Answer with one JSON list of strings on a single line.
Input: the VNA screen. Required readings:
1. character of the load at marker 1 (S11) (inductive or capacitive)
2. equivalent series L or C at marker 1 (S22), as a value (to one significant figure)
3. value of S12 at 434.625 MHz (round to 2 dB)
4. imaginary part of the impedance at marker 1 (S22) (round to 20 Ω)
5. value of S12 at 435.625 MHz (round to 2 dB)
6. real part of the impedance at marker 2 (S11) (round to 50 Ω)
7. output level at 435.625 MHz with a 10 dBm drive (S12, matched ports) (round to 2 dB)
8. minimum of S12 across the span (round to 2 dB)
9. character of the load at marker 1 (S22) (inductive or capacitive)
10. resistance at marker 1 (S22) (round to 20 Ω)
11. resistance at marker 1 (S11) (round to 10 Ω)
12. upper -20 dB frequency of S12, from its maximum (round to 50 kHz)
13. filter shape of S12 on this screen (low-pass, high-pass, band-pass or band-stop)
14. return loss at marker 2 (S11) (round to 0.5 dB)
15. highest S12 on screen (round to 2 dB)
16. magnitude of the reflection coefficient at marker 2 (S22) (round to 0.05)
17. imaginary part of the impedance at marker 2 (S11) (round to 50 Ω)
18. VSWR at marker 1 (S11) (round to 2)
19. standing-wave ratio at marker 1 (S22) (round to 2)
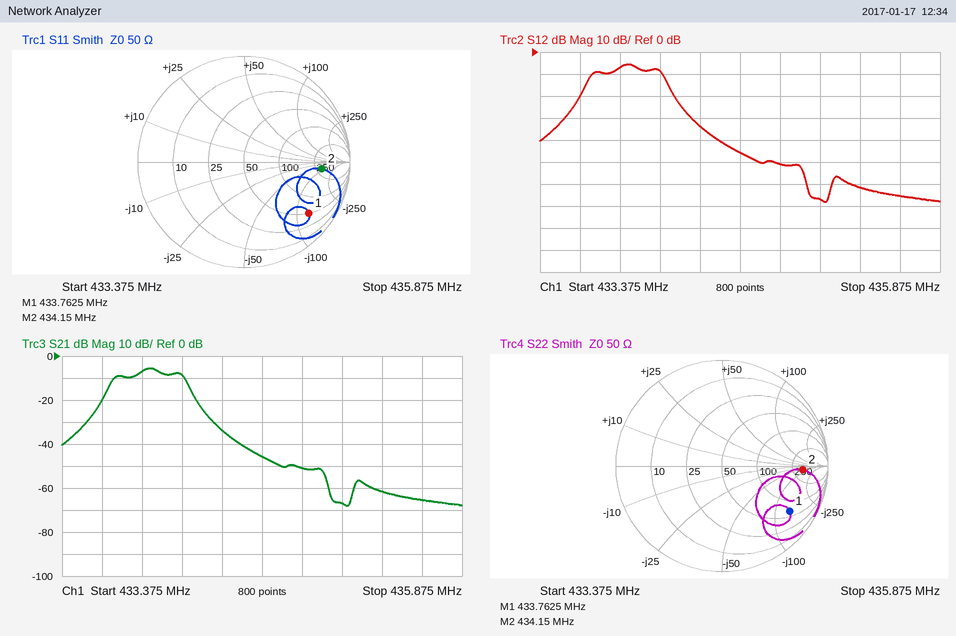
["capacitive", "3 pF", "-46 dB", "-140 Ω", "-66 dB", "300 Ω", "-56 dBm", "-68 dB", "capacitive", "60 Ω", "50 Ω", "434.25 MHz", "band-pass", "2.5 dB", "-6 dB", "0.75", "-100 Ω", "8", "8"]
